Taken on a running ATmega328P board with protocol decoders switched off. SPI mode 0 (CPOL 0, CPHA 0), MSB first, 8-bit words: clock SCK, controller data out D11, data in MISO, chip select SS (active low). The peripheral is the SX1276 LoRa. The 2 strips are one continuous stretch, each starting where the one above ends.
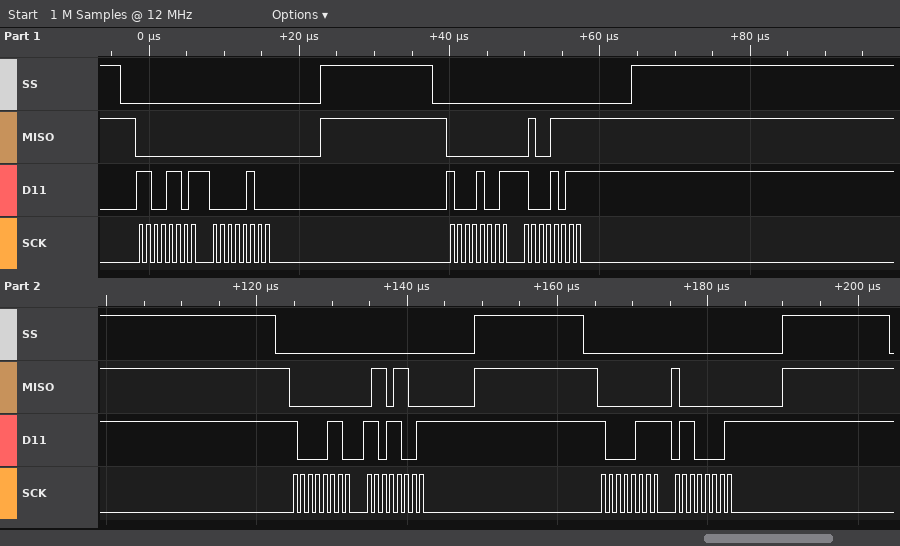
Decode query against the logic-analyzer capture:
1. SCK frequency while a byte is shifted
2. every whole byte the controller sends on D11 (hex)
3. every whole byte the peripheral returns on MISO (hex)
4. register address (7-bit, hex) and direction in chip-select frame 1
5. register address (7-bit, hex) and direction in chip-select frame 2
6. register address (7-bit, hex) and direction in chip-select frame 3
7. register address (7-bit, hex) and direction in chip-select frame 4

1 MHz
CD 04 89 8B 86 D9 87 61
00 00 00 4F 00 6C 00 80
0x4D write
0x09 write
0x06 write
0x07 write
